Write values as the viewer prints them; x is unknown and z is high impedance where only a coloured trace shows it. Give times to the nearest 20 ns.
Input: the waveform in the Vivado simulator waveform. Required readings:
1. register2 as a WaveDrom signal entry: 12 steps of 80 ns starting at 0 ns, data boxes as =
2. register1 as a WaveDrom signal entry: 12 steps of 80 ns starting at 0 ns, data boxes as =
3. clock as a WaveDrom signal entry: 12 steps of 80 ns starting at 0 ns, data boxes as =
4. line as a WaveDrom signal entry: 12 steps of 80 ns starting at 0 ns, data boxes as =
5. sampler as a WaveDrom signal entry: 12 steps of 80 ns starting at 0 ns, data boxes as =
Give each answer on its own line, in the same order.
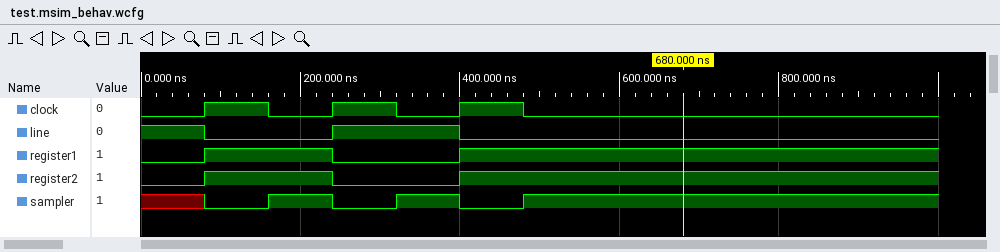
{name: 'register2', wave: '01.0.1......'}
{name: 'register1', wave: '01.0.1......'}
{name: 'clock', wave: '0101010.....'}
{name: 'line', wave: '10.1.0......'}
{name: 'sampler', wave: 'x010101.....'}
